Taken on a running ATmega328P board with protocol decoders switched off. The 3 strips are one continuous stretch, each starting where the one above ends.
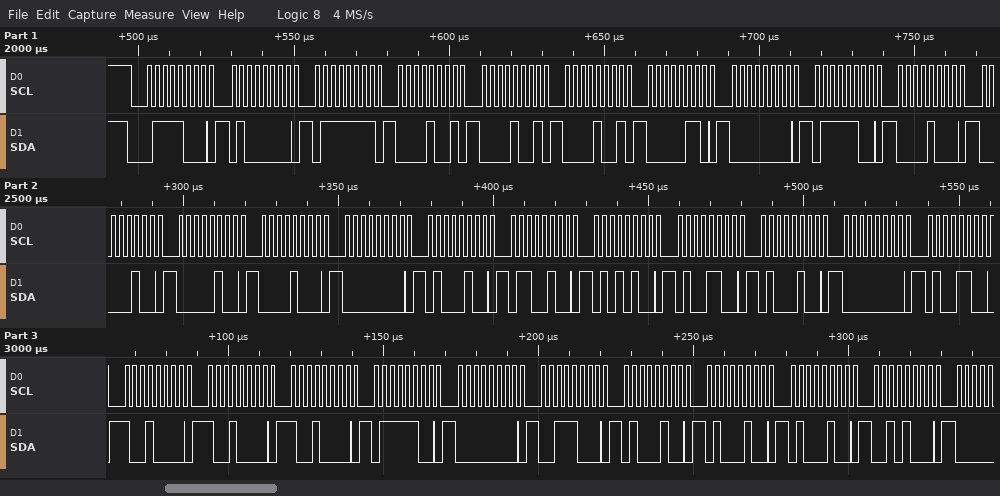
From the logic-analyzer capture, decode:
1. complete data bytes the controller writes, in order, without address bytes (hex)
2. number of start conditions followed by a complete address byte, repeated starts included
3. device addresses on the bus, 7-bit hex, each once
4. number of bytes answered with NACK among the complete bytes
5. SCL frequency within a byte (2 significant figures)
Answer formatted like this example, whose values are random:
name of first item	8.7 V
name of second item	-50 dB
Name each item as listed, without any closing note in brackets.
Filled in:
complete data bytes the controller writes, in order, without address bytes	40 7F 09 09 09 06 00 7C 08 04 04 08 00 44 64 54 4C 44 00 4C 90 90 90 7C 00 38 44 44 44 28
number of start conditions followed by a complete address byte, repeated starts included	1
device addresses on the bus, 7-bit hex, each once	0x3C
number of bytes answered with NACK among the complete bytes	0
SCL frequency within a byte	400 kHz
